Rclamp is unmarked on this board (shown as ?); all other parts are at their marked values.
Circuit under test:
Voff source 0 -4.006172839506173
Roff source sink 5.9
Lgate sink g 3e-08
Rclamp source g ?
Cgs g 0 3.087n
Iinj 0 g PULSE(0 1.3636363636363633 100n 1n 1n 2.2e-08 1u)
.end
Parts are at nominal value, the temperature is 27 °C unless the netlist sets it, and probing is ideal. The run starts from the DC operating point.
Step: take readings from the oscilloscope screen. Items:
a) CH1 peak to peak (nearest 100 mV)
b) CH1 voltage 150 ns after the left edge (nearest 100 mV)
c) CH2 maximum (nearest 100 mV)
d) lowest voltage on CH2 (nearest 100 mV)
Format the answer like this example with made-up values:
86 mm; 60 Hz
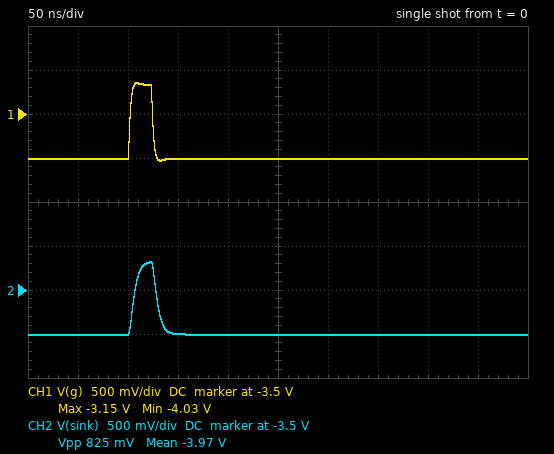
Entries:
900 mV; -4.0 V; -3.2 V; -4.0 V
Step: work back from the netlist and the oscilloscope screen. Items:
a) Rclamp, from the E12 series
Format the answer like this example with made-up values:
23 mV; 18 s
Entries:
0.68 Ω
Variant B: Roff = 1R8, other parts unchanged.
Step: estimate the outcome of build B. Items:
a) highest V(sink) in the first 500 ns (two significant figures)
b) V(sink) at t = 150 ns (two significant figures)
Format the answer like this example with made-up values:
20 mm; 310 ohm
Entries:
-3.4 V; -3.9 V
